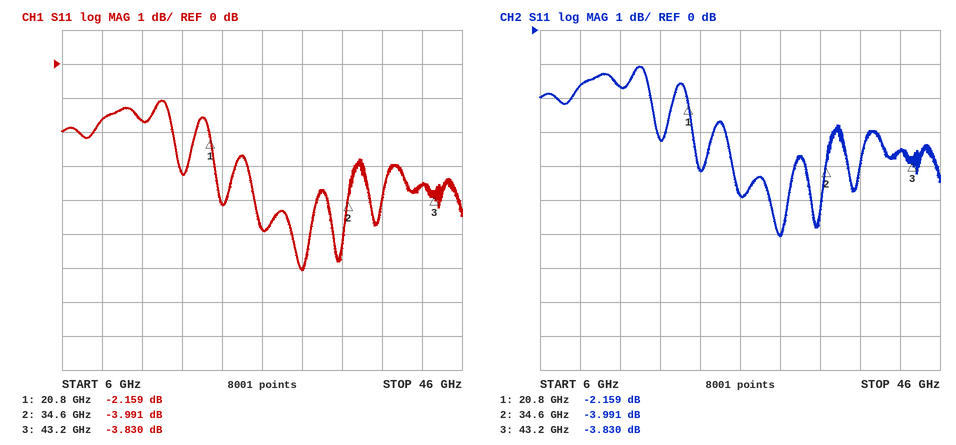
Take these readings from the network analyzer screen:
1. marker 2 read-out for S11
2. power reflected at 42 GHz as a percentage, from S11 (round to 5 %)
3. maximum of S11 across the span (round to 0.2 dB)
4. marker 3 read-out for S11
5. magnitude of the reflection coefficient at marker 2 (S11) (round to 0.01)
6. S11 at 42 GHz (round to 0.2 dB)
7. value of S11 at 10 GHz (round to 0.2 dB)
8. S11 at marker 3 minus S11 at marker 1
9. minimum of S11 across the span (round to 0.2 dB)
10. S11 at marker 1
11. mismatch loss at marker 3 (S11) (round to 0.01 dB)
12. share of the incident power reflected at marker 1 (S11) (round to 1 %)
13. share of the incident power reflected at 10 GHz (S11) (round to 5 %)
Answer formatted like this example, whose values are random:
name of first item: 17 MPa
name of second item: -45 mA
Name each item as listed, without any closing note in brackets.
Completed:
marker 2 read-out for S11: -3.991 dB
power reflected at 42 GHz as a percentage, from S11: 45 %
maximum of S11 across the span: -1.0 dB
marker 3 read-out for S11: -3.830 dB
magnitude of the reflection coefficient at marker 2 (S11): 0.63
S11 at 42 GHz: -3.6 dB
value of S11 at 10 GHz: -1.6 dB
S11 at marker 3 minus S11 at marker 1: -1.671 dB
minimum of S11 across the span: -6.0 dB
S11 at marker 1: -2.159 dB
mismatch loss at marker 3 (S11): 2.32 dB
share of the incident power reflected at marker 1 (S11): 61 %
share of the incident power reflected at 10 GHz (S11): 70 %
